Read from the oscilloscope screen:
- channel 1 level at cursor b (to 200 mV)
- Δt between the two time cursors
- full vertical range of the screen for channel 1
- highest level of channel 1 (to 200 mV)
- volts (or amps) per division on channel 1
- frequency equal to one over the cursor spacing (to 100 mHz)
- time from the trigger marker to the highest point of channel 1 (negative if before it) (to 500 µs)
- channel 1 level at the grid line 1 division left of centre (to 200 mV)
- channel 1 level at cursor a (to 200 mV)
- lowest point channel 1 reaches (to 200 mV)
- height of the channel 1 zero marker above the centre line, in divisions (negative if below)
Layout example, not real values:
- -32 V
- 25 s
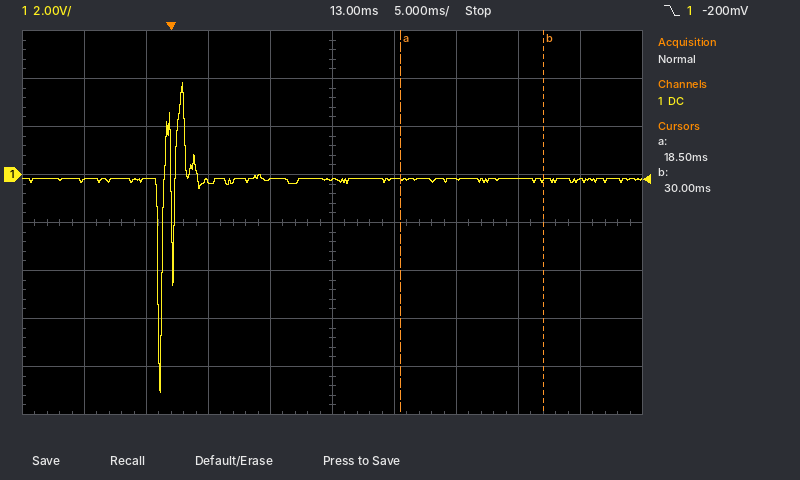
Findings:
- -200 mV
- 11.5 ms
- 16 V
- 3.8 V
- 2 V
- 87.0 Hz
- +1.0 ms
- -200 mV
- -200 mV
- -9.0 V
- +1.0 div
